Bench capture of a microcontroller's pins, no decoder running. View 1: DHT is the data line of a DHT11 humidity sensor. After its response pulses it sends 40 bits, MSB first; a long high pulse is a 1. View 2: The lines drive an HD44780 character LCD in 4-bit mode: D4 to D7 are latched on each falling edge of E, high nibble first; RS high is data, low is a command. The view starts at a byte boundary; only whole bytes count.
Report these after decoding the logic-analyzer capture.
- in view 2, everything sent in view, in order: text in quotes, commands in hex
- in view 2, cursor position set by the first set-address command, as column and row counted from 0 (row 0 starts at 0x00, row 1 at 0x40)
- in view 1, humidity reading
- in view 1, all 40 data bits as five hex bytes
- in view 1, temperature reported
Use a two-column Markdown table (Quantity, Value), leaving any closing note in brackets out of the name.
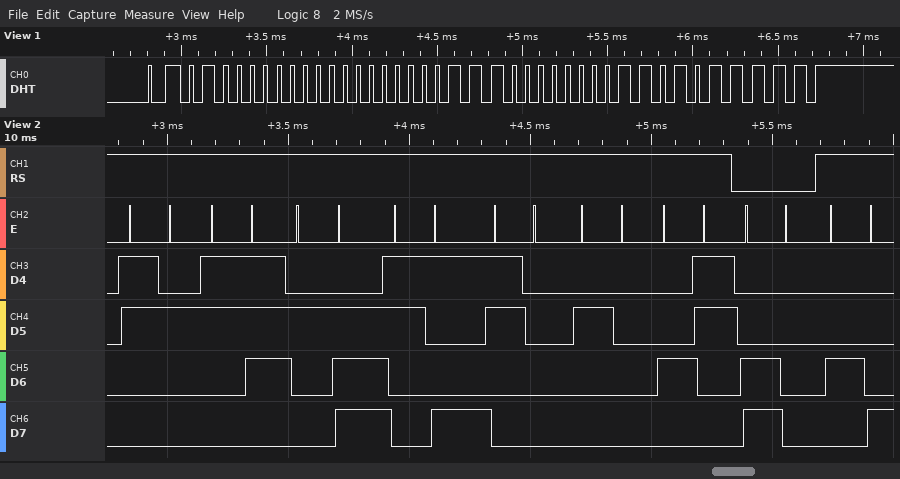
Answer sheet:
| Quantity | Value |
|---|---|
| in view 2, everything sent in view, in order: text in quotes, commands in hex | "27.90 C" 0xC0 "H" |
| in view 2, cursor position set by the first set-address command, as column and row counted from 0 | column 0, row 1 |
| in view 1, humidity reading | 64 % |
| in view 1, all 40 data bits as five hex bytes | 40 00 1C 03 5F |
| in view 1, temperature reported | 28.3 °C |
